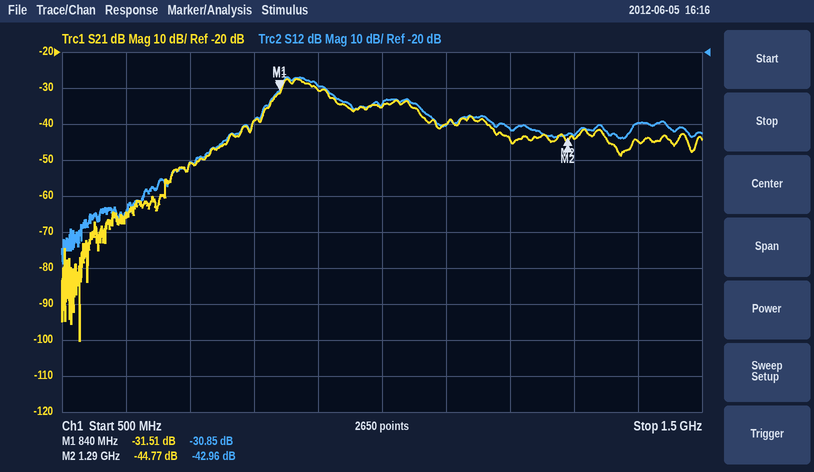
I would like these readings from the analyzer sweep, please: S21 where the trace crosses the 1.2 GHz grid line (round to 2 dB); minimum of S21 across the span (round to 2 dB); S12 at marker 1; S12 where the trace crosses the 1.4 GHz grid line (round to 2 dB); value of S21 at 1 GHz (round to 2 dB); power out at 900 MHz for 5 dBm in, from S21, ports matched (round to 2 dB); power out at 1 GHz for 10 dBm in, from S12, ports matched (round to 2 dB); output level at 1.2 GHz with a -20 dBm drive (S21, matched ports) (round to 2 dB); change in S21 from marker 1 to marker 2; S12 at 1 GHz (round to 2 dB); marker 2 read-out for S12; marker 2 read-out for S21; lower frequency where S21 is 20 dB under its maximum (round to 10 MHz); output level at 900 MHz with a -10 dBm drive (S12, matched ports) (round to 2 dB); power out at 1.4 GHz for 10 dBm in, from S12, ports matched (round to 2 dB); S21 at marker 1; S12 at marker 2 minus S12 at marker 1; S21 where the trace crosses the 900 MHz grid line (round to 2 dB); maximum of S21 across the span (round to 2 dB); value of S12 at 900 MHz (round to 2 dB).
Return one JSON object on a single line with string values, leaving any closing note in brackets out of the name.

{"S21 where the trace crosses the 1.2 GHz grid line": "-44 dB", "minimum of S21 across the span": "-100 dB", "S12 at marker 1": "-30.85 dB", "S12 where the trace crosses the 1.4 GHz grid line": "-40 dB", "value of S21 at 1 GHz": "-36 dB", "power out at 900 MHz for 5 dBm in, from S21, ports matched": "-26 dBm", "power out at 1 GHz for 10 dBm in, from S12, ports matched": "-24 dBm", "output level at 1.2 GHz with a -20 dBm drive (S21, matched ports)": "-64 dBm", "change in S21 from marker 1 to marker 2": "-13.26 dB", "S12 at 1 GHz": "-34 dB", "marker 2 read-out for S12": "-42.96 dB", "marker 2 read-out for S21": "-44.77 dB", "lower frequency where S21 is 20 dB under its maximum": "730 MHz", "output level at 900 MHz with a -10 dBm drive (S12, matched ports)": "-40 dBm", "power out at 1.4 GHz for 10 dBm in, from S12, ports matched": "-30 dBm", "S21 at marker 1": "-31.51 dB", "S12 at marker 2 minus S12 at marker 1": "-12.11 dB", "S21 where the trace crosses the 900 MHz grid line": "-30 dB", "maximum of S21 across the span": "-28 dB", "value of S12 at 900 MHz": "-30 dB"}
